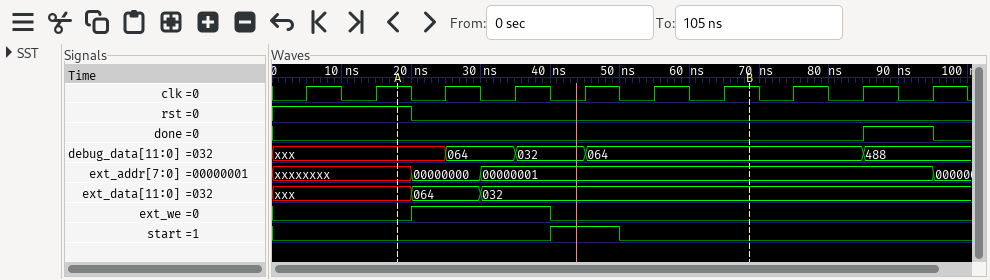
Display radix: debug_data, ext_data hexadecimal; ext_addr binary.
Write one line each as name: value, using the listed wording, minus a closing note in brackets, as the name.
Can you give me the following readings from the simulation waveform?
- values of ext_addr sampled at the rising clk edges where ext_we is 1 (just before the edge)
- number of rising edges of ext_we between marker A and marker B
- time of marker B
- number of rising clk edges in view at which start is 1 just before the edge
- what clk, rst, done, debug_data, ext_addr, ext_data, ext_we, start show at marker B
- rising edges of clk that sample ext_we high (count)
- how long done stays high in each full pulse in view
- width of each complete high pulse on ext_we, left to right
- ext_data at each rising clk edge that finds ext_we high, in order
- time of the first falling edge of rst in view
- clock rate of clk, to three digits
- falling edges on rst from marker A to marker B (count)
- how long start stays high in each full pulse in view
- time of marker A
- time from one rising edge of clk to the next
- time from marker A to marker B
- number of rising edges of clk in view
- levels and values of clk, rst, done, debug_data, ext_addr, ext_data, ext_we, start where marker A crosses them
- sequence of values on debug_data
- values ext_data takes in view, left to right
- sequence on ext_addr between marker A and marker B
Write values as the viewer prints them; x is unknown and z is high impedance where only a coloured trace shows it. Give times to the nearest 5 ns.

values of ext_addr sampled at the rising clk edges where ext_we is 1: 00000000, 00000001
number of rising edges of ext_we between marker A and marker B: 1
time of marker B: 70 ns
number of rising clk edges in view at which start is 1 just before the edge: 1
what clk, rst, done, debug_data, ext_addr, ext_data, ext_we, start show at marker B: clk=1, rst=0, done=0, debug_data=064, ext_addr=00000001, ext_data=032, ext_we=0, start=0
rising edges of clk that sample ext_we high: 2
how long done stays high in each full pulse in view: 10 ns
width of each complete high pulse on ext_we, left to right: 20 ns
ext_data at each rising clk edge that finds ext_we high, in order: 064, 032
time of the first falling edge of rst in view: 20 ns
clock rate of clk, to three digits: 100 MHz
falling edges on rst from marker A to marker B: 1
how long start stays high in each full pulse in view: 10 ns
time of marker A: 20 ns
time from one rising edge of clk to the next: 10 ns
time from marker A to marker B: 50 ns
number of rising edges of clk in view: 10
levels and values of clk, rst, done, debug_data, ext_addr, ext_data, ext_we, start where marker A crosses them: clk=1, rst=1, done=0, debug_data=xxx, ext_addr=xxxxxxxx, ext_data=xxx, ext_we=0, start=0
sequence of values on debug_data: xxx, 064, 032, 064, 488
values ext_data takes in view, left to right: xxx, 064, 032
sequence on ext_addr between marker A and marker B: xxxxxxxx, 00000000, 00000001
